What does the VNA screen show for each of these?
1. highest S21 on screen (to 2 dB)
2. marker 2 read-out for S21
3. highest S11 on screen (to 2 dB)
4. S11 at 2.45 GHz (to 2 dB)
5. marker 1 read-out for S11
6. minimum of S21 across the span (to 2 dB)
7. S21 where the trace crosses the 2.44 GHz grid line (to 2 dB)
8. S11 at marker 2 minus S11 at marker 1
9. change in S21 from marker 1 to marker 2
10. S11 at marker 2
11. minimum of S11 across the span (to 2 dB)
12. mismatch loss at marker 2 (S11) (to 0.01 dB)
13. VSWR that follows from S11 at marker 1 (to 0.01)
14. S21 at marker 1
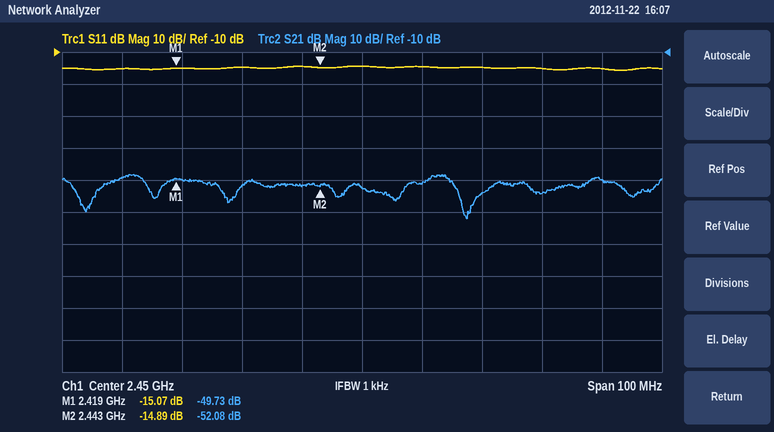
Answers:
-48 dB
-52.08 dB
-14 dB
-14 dB
-15.07 dB
-62 dB
-52 dB
0.18 dB
-2.35 dB
-14.89 dB
-16 dB
0.14 dB
1.43
-49.73 dB
